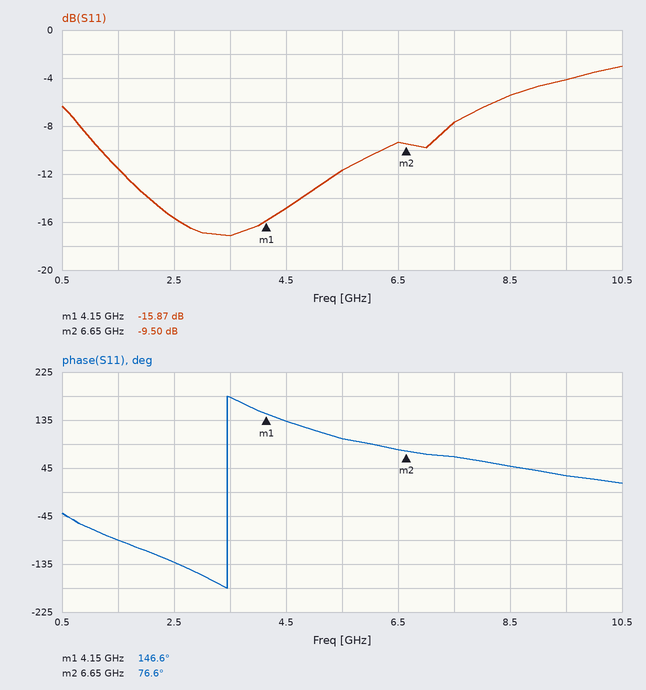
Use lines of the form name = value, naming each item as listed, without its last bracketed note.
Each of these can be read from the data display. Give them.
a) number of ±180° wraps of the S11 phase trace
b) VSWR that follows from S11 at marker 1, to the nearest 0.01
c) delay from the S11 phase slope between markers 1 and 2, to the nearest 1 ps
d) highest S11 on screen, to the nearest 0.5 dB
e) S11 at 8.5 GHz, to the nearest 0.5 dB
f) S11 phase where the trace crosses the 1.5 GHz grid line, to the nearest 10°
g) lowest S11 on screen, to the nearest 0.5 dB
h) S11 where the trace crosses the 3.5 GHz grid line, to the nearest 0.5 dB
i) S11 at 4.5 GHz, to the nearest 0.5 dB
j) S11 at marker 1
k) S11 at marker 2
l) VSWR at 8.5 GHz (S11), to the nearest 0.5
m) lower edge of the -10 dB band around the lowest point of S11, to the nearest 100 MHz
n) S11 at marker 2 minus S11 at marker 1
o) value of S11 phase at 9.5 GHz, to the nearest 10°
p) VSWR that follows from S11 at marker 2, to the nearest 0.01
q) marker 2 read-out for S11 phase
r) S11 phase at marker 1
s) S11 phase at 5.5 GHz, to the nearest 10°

number of ±180° wraps of the S11 phase trace = 1
VSWR that follows from S11 at marker 1, to the nearest 0.01 = 1.38
delay from the S11 phase slope between markers 1 and 2, to the nearest 1 ps = 78 ps
highest S11 on screen, to the nearest 0.5 dB = -3.0 dB
S11 at 8.5 GHz, to the nearest 0.5 dB = -5.5 dB
S11 phase where the trace crosses the 1.5 GHz grid line, to the nearest 10° = -90°
lowest S11 on screen, to the nearest 0.5 dB = -17.0 dB
S11 where the trace crosses the 3.5 GHz grid line, to the nearest 0.5 dB = -17.0 dB
S11 at 4.5 GHz, to the nearest 0.5 dB = -15.0 dB
S11 at marker 1 = -15.87 dB
S11 at marker 2 = -9.50 dB
VSWR at 8.5 GHz (S11), to the nearest 0.5 = 3.5
lower edge of the -10 dB band around the lowest point of S11, to the nearest 100 MHz = 1.2 GHz
S11 at marker 2 minus S11 at marker 1 = 6.37 dB
value of S11 phase at 9.5 GHz, to the nearest 10° = 30°
VSWR that follows from S11 at marker 2, to the nearest 0.01 = 2.01
marker 2 read-out for S11 phase = 76.6°
S11 phase at marker 1 = 146.6°
S11 phase at 5.5 GHz, to the nearest 10° = 100°
